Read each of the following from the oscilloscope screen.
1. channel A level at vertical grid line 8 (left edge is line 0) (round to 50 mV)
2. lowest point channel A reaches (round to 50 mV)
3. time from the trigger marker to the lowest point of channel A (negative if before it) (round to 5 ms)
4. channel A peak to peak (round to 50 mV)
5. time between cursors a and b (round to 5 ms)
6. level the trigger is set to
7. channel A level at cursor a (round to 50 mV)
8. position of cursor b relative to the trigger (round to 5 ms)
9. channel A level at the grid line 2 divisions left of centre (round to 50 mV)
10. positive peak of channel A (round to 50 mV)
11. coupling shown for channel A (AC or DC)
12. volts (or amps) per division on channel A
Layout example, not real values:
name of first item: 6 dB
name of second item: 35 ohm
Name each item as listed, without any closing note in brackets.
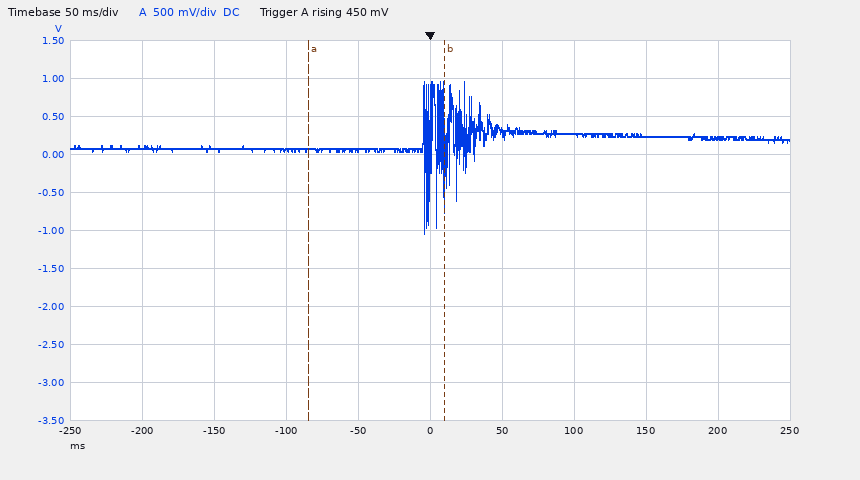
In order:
channel A level at vertical grid line 8 (left edge is line 0): 250 mV
lowest point channel A reaches: -1.05 V
time from the trigger marker to the lowest point of channel A (negative if before it): -5 ms
channel A peak to peak: 2.00 V
time between cursors a and b: 95 ms
level the trigger is set to: 450 mV
channel A level at cursor a: 50 mV
position of cursor b relative to the trigger: +10 ms
channel A level at the grid line 2 divisions left of centre: 50 mV
positive peak of channel A: 950 mV
coupling shown for channel A: DC
volts (or amps) per division on channel A: 500 mV
